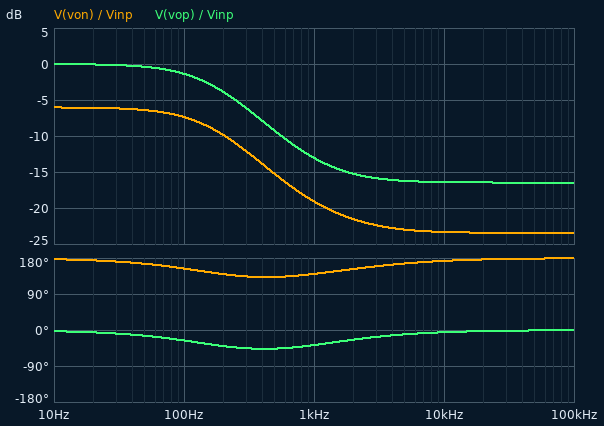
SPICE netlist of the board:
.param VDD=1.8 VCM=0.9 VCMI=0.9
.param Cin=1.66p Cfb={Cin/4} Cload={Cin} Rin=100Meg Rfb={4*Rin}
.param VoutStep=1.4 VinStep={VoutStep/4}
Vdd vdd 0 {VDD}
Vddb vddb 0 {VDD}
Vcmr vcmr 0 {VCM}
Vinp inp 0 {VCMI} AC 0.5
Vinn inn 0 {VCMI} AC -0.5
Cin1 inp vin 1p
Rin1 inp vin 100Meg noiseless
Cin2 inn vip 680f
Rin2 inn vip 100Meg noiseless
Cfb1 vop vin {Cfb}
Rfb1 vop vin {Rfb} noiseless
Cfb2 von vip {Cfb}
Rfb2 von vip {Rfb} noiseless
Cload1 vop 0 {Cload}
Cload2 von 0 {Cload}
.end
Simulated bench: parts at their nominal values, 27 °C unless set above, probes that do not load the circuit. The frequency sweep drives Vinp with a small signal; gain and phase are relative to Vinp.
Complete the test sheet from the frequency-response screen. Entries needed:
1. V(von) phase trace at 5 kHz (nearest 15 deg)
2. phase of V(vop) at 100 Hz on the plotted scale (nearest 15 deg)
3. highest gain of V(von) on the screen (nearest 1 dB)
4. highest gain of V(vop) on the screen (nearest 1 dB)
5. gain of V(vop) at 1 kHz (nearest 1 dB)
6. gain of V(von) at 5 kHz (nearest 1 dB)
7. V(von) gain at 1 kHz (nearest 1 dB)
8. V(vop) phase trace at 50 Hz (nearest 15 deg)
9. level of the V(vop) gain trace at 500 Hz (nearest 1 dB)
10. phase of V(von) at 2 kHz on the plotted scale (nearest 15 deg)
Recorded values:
165 deg
-30 deg
-6 dB
0 dB
-13 dB
-23 dB
-19 dB
-15 deg
-9 dB
150 deg
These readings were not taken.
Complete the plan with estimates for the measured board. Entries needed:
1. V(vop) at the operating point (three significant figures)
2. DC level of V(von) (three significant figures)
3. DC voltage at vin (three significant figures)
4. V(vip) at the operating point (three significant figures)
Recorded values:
900 mV
900 mV
900 mV
900 mV
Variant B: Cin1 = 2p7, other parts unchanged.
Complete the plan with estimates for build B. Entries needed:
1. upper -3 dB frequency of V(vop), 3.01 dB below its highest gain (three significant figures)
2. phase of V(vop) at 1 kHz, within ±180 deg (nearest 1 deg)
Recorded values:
162 Hz
-33 deg
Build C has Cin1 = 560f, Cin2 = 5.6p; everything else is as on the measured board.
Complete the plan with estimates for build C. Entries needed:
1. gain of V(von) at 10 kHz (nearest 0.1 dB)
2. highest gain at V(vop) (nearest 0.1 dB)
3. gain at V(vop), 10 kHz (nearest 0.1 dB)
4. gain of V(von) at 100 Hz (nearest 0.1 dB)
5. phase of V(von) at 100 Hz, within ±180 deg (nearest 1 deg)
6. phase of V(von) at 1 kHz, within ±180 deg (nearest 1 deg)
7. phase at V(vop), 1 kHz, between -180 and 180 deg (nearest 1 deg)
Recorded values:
-20.5 dB
0 dB
-17.8 dB
-7.5 dB
155 deg
148 deg
-41 deg
